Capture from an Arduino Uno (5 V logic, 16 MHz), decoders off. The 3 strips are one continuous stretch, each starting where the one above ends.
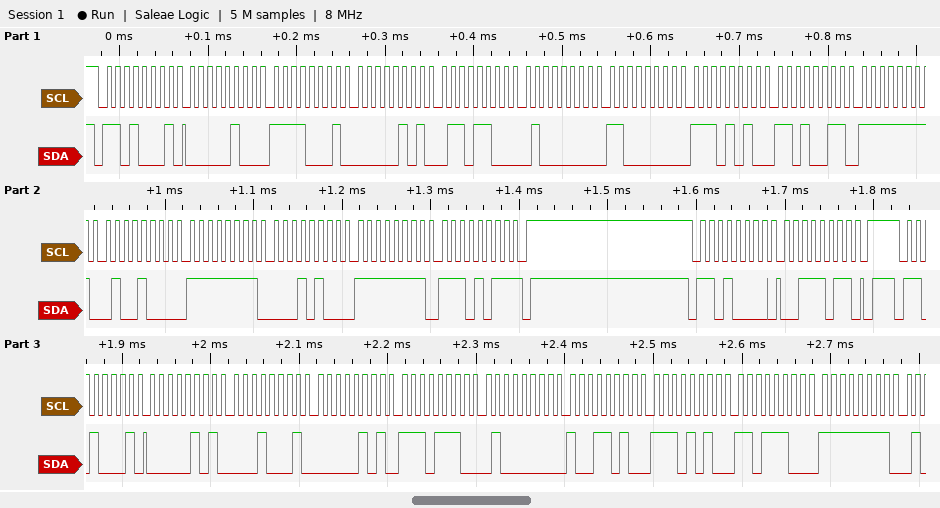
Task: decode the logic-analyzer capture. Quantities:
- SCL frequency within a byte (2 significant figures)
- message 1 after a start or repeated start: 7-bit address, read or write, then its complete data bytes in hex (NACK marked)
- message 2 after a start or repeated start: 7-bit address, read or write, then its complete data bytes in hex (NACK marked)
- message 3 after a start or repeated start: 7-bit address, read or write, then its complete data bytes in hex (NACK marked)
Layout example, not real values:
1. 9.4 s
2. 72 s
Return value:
1. 100 kHz
2. 0x68 read: 04 F1 05 6C 40 C0 EA D3 FF 48 FF 14 FF EB NACK
3. 0x68 write: 3B
4. 0x68 read: 05 11 05 EE 40 9A EA DC FF
